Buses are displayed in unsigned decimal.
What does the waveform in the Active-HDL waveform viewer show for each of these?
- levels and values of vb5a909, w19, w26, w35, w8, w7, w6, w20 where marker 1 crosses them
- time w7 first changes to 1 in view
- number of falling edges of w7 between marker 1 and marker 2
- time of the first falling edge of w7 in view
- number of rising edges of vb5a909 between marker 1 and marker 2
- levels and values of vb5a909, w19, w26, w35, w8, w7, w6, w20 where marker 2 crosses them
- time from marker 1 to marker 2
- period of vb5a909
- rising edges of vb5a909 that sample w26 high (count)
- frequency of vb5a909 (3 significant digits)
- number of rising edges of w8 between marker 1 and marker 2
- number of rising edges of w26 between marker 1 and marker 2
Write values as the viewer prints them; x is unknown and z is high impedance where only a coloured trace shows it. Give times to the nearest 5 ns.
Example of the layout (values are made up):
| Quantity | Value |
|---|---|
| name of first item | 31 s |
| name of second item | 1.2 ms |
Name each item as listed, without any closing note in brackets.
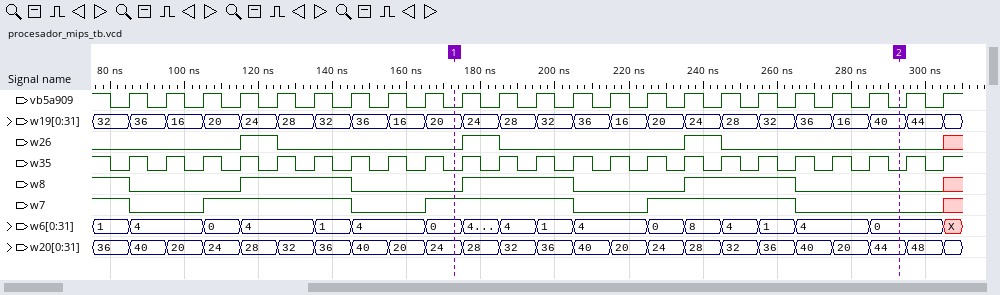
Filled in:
| Quantity | Value |
|---|---|
| levels and values of vb5a909, w19, w26, w35, w8, w7, w6, w20 where marker 1 crosses them | vb5a909=0, w19=20, w26=0, w35=0, w8=0, w7=1, w6=0, w20=24 |
| time w7 first changes to 1 in view | 105 ns |
| number of falling edges of w7 between marker 1 and marker 2 | 2 |
| time of the first falling edge of w7 in view | 85 ns |
| number of rising edges of vb5a909 between marker 1 and marker 2 | 12 |
| levels and values of vb5a909, w19, w26, w35, w8, w7, w6, w20 where marker 2 crosses them | vb5a909=0, w19=40, w26=0, w35=0, w8=0, w7=0, w6=0, w20=44 |
| time from marker 1 to marker 2 | 120 ns |
| period of vb5a909 | 10 ns |
| rising edges of vb5a909 that sample w26 high | 3 |
| frequency of vb5a909 | 100 MHz |
| number of rising edges of w8 between marker 1 and marker 2 | 2 |
| number of rising edges of w26 between marker 1 and marker 2 | 2 |
